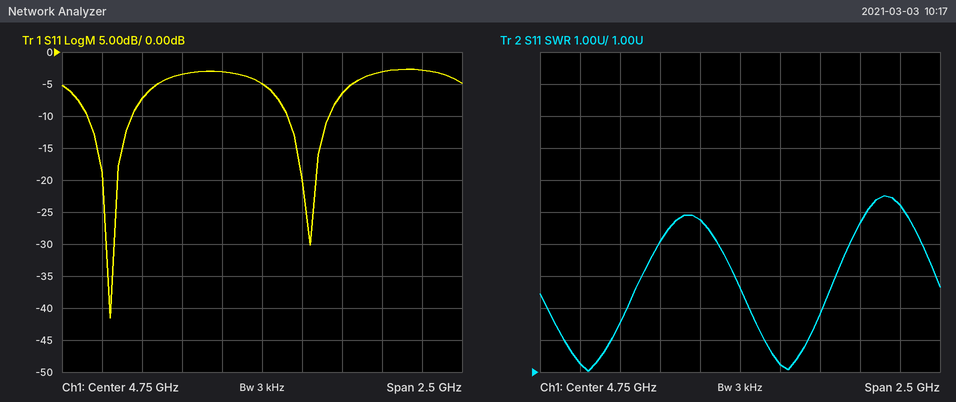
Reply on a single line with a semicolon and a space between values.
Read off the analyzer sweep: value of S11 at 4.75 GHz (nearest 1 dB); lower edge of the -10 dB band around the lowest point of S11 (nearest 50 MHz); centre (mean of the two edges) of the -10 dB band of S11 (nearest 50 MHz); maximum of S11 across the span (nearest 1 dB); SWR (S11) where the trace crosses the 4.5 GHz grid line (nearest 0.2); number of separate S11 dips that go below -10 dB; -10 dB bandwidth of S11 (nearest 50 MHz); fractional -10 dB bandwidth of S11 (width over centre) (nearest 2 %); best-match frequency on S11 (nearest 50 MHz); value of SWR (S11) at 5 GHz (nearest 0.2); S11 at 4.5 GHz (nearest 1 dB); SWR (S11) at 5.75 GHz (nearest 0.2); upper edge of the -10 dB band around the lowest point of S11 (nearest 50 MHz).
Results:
-5 dB; 3.65 GHz; 3.80 GHz; -3 dB; 5.8; 2; 300 MHz; 8 %; 3.80 GHz; 1.2; -3 dB; 6.2; 3.95 GHz
